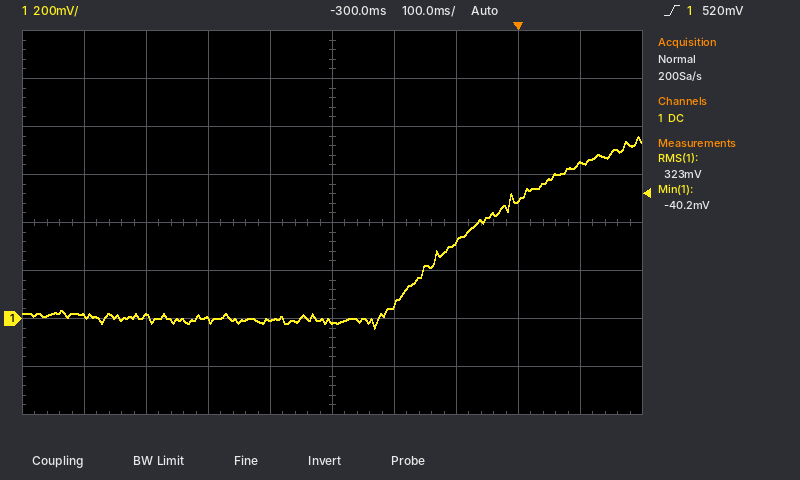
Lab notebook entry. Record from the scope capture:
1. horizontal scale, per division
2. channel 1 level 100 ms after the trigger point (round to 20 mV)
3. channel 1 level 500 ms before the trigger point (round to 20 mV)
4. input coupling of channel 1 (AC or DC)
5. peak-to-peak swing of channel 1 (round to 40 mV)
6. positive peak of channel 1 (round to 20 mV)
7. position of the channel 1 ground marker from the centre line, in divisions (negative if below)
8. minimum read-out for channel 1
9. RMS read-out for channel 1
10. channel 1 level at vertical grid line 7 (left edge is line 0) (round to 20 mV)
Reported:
100 ms
640 mV
0 mV
DC
800 mV
760 mV
-2.0 div
-40.2 mV
323 mV
320 mV
